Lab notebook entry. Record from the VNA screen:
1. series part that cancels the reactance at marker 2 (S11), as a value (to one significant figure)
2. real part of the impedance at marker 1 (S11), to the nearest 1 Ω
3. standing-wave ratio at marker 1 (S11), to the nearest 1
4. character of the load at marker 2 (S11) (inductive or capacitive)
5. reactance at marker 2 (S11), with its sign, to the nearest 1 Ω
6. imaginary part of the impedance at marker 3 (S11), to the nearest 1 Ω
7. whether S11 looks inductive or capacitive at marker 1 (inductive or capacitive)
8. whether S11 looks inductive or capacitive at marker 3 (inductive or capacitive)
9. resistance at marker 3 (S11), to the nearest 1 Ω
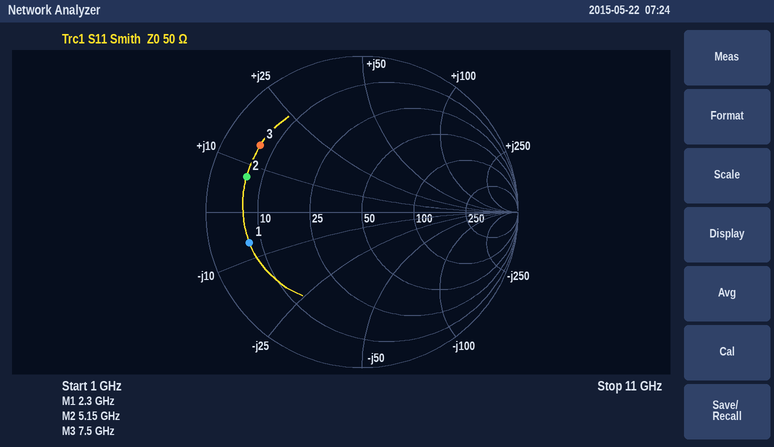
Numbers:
4 pF
7 Ω
7
inductive
+7 Ω
+15 Ω
capacitive
inductive
7 Ω
